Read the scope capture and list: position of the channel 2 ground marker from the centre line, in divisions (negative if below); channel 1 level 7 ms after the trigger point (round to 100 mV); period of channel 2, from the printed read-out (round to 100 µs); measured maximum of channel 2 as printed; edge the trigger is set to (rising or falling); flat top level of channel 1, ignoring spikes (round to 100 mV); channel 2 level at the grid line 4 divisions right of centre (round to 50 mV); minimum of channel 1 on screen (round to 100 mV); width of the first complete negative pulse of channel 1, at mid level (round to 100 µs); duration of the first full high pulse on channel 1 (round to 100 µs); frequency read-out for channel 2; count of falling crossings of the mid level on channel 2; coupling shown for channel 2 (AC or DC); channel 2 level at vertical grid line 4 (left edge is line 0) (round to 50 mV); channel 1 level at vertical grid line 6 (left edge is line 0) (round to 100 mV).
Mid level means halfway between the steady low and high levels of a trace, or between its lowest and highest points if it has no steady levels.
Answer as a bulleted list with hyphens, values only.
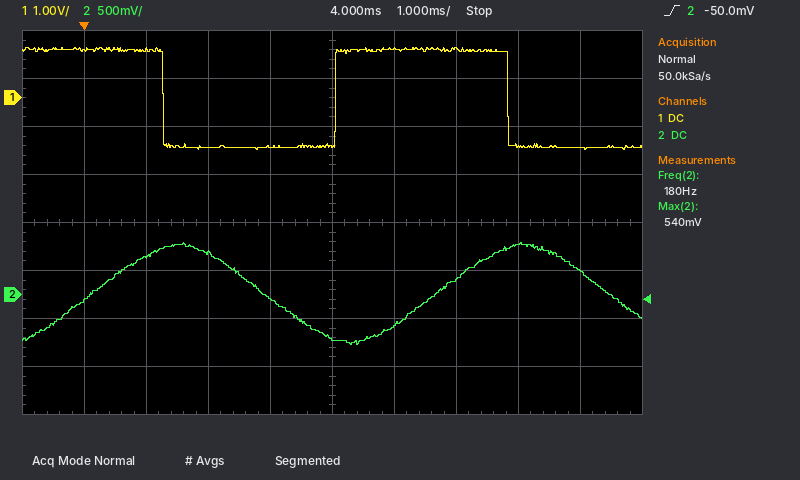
- -1.5 div
- -1.0 V
- 5.6 ms
- 540 mV
- rising
- 1.0 V
- 250 mV
- -1.1 V
- 2.8 ms
- 2.8 ms
- 180 Hz
- 2
- DC
- -50 mV
- 1.0 V
